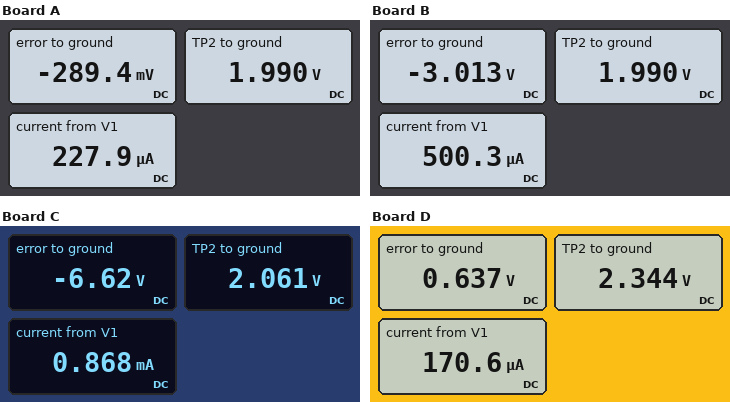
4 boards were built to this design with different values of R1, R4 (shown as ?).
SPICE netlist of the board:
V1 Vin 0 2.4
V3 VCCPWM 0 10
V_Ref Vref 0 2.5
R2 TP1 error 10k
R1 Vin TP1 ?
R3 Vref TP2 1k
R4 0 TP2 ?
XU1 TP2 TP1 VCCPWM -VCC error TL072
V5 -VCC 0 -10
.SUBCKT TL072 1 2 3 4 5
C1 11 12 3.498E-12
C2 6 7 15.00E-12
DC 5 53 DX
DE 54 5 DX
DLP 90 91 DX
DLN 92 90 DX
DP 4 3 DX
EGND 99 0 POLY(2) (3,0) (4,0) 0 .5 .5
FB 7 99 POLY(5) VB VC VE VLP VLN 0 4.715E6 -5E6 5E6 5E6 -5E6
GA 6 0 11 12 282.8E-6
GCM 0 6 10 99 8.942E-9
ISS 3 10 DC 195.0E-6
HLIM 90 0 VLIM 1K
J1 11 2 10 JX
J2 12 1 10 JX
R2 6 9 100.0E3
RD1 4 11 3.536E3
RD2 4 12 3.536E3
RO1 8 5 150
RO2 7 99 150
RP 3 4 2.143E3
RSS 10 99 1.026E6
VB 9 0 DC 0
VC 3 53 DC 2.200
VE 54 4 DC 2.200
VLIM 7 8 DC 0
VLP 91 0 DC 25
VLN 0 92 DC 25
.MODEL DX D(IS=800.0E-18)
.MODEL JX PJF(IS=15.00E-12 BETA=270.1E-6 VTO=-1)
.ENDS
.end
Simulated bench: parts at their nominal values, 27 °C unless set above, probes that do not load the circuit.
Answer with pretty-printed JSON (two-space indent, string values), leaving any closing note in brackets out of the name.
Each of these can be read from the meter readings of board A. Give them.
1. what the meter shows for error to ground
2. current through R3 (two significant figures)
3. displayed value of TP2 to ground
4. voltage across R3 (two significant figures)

{
  "what the meter shows for error to ground": "-289.4 mV",
  "current through R3": "510 µA",
  "displayed value of TP2 to ground": "1.990 V",
  "voltage across R3": "510 mV"
}
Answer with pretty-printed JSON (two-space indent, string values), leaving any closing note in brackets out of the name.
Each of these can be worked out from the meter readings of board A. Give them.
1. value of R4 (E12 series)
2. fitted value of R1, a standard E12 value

{
  "value of R4": "3.9 kΩ",
  "fitted value of R1, a standard E12 value": "1.8 kΩ"
}
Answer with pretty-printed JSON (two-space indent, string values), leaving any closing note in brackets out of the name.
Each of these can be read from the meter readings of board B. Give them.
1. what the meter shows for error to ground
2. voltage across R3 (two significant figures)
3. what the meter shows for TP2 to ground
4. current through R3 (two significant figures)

{
  "what the meter shows for error to ground": "-3.013 V",
  "voltage across R3": "510 mV",
  "what the meter shows for TP2 to ground": "1.990 V",
  "current through R3": "510 µA"
}
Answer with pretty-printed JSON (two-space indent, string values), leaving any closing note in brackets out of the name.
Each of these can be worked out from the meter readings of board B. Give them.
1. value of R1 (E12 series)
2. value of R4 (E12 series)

{
  "value of R1": "820 Ω",
  "value of R4": "3.9 kΩ"
}
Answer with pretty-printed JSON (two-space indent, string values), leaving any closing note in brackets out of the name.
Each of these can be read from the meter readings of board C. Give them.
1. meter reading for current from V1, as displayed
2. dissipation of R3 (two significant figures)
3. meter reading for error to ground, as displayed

{
  "meter reading for current from V1, as displayed": "0.868 mA",
  "dissipation of R3": "190 µW",
  "meter reading for error to ground, as displayed": "-6.62 V"
}
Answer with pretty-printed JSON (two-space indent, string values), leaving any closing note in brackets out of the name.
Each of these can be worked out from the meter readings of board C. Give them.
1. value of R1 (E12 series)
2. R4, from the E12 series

{
  "value of R1": "390 Ω",
  "R4, from the E12 series": "4.7 kΩ"
}
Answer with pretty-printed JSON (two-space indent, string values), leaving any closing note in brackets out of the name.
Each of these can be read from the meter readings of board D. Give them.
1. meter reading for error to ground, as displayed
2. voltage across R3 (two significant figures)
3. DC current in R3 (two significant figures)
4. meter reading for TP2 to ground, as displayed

{
  "meter reading for error to ground, as displayed": "0.637 V",
  "voltage across R3": "160 mV",
  "DC current in R3": "160 µA",
  "meter reading for TP2 to ground, as displayed": "2.344 V"
}
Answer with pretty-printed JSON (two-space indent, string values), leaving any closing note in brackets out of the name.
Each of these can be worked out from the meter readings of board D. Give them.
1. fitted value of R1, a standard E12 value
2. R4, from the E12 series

{
  "fitted value of R1, a standard E12 value": "330 Ω",
  "R4, from the E12 series": "15 kΩ"
}
